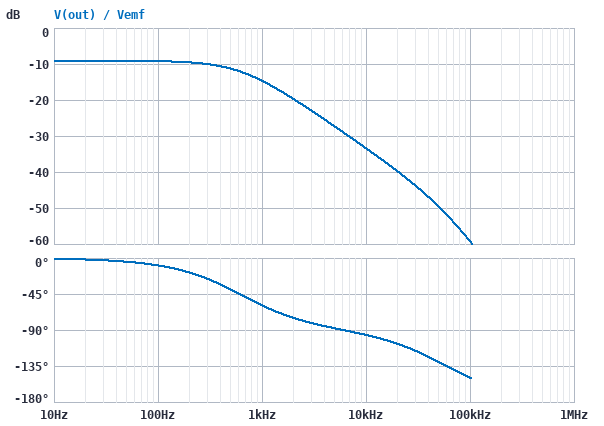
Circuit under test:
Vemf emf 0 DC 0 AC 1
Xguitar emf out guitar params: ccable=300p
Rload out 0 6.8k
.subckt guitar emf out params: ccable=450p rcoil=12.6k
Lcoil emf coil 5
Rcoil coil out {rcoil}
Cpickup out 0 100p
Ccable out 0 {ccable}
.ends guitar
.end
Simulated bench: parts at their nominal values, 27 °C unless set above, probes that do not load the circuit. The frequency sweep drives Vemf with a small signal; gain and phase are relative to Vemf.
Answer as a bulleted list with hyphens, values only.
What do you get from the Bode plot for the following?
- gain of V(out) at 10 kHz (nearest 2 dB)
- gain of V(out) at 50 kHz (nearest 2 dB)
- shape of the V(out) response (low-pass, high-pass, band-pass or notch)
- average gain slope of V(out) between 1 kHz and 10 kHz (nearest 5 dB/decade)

- -34 dB
- -50 dB
- low-pass
- -20 dB/decade
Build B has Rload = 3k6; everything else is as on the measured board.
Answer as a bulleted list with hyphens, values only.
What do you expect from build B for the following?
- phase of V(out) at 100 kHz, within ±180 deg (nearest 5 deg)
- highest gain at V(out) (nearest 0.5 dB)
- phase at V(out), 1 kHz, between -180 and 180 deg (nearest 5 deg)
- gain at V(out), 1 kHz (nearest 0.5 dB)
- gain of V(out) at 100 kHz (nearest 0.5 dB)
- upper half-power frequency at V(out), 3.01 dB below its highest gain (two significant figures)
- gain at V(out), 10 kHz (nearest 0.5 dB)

- -130 deg
- -13.0 dB
- -65 deg
- -20.0 dB
- -61.5 dB
- 520 Hz
- -39.0 dB
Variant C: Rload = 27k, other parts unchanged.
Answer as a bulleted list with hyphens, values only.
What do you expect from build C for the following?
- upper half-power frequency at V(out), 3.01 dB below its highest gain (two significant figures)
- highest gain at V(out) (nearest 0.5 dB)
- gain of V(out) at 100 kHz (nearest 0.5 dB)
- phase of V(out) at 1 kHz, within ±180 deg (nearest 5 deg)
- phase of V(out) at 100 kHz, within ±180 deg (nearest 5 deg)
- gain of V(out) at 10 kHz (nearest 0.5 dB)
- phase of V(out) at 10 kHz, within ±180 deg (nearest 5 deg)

- 1.3 kHz
- -3.5 dB
- -58.0 dB
- -40 deg
- -170 deg
- -22.5 dB
- -120 deg
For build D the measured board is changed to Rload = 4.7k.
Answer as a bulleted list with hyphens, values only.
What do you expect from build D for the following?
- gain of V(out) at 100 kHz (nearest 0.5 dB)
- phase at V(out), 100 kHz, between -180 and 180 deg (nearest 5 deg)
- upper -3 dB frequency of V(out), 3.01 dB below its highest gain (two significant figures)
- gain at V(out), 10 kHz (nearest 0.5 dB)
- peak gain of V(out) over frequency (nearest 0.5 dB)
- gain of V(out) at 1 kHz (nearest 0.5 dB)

- -60.5 dB
- -140 deg
- 550 Hz
- -36.5 dB
- -11.5 dB
- -17.5 dB
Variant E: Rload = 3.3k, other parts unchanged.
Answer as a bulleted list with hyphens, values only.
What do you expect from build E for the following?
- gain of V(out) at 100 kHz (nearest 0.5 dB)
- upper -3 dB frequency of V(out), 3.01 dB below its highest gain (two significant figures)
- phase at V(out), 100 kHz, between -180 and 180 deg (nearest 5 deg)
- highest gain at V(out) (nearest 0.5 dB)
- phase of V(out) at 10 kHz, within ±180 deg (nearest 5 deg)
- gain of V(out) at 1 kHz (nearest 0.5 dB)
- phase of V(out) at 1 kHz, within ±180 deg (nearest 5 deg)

- -62.0 dB
- 510 Hz
- -130 deg
- -13.5 dB
- -90 deg
- -20.5 dB
- -65 deg
